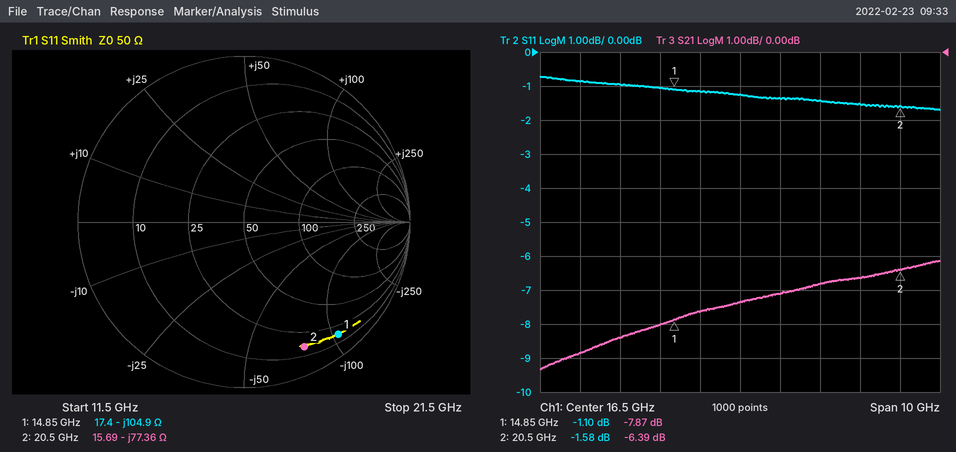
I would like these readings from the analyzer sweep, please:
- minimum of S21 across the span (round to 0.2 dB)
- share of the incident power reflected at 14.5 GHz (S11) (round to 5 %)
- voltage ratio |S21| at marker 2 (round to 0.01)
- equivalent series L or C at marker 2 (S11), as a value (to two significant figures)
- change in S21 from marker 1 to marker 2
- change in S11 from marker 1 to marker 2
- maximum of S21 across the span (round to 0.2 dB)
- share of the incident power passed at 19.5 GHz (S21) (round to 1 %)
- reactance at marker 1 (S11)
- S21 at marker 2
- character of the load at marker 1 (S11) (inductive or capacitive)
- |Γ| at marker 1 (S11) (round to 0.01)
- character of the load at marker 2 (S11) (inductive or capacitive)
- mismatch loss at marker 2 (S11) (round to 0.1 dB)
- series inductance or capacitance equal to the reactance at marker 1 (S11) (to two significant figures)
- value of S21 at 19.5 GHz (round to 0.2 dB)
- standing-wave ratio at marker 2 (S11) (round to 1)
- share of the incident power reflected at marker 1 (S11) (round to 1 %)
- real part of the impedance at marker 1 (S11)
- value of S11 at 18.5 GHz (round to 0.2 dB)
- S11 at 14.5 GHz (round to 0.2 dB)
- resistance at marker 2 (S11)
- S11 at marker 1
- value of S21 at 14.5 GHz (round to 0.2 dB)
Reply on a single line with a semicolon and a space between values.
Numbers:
-9.4 dB; 80 %; 0.48; 100 fF; 1.48 dB; -0.48 dB; -6.2 dB; 22 %; -104.9 Ω; -6.39 dB; capacitive; 0.88; capacitive; 5.2 dB; 100 fF; -6.6 dB; 11; 78 %; 17.4 Ω; -1.4 dB; -1.0 dB; 15.69 Ω; -1.10 dB; -8.0 dB
